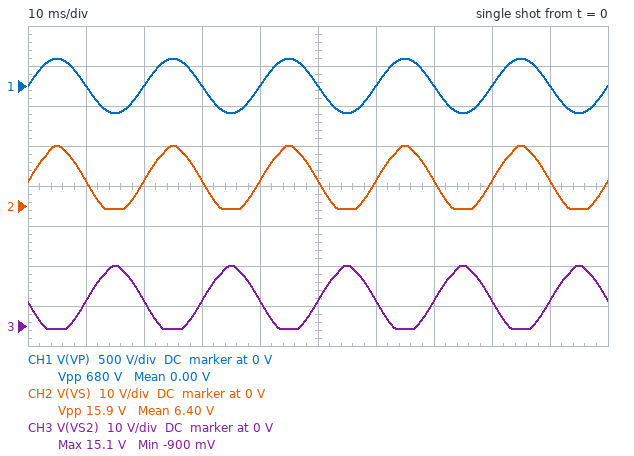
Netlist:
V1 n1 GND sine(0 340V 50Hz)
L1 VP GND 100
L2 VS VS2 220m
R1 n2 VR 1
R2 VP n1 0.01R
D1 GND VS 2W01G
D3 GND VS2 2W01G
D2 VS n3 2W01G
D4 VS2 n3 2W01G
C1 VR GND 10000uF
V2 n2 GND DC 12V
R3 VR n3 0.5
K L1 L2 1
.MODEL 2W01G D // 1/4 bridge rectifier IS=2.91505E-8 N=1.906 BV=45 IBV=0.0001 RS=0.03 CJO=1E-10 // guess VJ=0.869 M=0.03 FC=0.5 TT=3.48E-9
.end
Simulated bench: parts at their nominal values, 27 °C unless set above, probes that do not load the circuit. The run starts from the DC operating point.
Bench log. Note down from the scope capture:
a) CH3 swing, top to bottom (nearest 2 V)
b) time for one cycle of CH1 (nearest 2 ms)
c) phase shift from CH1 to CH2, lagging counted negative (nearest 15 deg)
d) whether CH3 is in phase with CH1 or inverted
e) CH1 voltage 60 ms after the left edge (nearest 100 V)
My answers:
16 V
20 ms
0 deg
inverted
0 V
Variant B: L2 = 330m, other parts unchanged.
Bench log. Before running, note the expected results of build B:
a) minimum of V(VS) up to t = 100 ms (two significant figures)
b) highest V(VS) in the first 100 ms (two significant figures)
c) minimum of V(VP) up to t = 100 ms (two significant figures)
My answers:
-890 mV
19 V
-340 V
